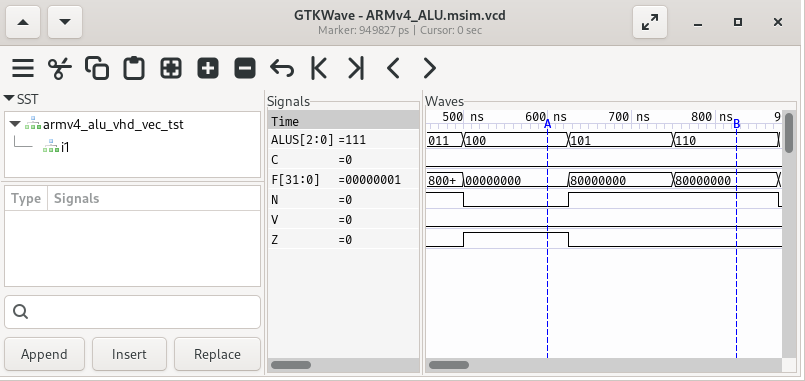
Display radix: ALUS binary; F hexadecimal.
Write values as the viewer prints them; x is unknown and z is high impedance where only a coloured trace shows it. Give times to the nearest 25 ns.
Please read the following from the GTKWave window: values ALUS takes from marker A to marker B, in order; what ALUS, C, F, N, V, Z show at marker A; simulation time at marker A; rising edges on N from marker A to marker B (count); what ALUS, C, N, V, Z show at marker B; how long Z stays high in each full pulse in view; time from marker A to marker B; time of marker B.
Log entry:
100, 101, 110
ALUS=100, C=0, F=00000000, N=0, V=0, Z=1
600 ns
1
ALUS=110, C=0, N=1, V=0, Z=0
125 ns
225 ns
825 ns
